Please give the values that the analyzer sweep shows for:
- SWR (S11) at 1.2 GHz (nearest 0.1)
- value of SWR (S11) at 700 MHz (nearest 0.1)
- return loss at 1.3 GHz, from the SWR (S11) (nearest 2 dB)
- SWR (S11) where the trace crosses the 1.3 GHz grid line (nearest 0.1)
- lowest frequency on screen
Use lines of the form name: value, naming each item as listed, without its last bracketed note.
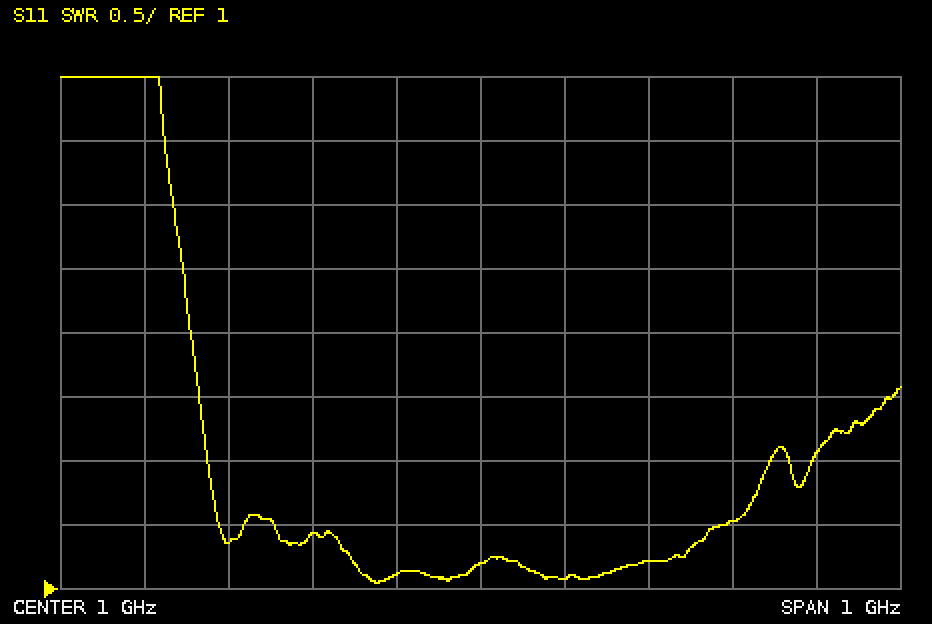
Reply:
SWR (S11) at 1.2 GHz: 1.2
value of SWR (S11) at 700 MHz: 1.4
return loss at 1.3 GHz, from the SWR (S11): 14 dB
SWR (S11) where the trace crosses the 1.3 GHz grid line: 1.5
lowest frequency on screen: 500 MHz
